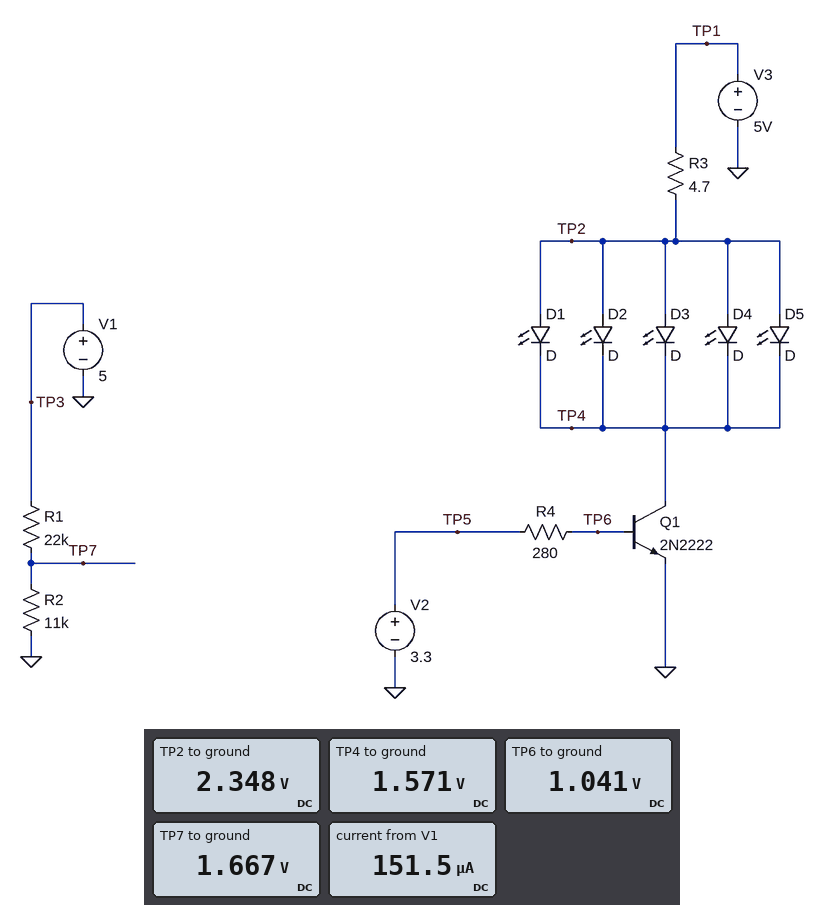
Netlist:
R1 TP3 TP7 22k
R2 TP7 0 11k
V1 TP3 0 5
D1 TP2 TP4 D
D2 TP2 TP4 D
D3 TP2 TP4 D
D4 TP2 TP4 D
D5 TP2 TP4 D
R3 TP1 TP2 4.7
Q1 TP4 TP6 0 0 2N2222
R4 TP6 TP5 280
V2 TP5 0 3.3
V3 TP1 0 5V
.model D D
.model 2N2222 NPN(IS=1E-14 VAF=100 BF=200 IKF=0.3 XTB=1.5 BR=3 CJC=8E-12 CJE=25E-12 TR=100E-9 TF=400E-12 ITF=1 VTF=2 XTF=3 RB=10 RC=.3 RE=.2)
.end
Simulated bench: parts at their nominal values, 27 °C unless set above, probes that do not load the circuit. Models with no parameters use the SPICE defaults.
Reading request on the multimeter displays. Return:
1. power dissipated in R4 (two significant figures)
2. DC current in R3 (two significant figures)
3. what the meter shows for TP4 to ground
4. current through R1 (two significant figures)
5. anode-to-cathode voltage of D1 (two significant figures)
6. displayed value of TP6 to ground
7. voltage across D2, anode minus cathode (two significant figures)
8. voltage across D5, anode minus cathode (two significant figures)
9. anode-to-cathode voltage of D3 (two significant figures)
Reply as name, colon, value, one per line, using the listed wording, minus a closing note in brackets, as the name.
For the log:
power dissipated in R4: 18 mW
DC current in R3: 560 mA
what the meter shows for TP4 to ground: 1.571 V
current through R1: 150 µA
anode-to-cathode voltage of D1: 780 mV
displayed value of TP6 to ground: 1.041 V
voltage across D2, anode minus cathode: 780 mV
voltage across D5, anode minus cathode: 780 mV
anode-to-cathode voltage of D3: 780 mV
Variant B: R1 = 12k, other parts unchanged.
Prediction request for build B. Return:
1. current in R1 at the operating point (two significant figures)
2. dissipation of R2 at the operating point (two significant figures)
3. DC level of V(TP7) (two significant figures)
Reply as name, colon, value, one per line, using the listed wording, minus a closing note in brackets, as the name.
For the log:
current in R1 at the operating point: 220 µA
dissipation of R2 at the operating point: 520 µW
DC level of V(TP7): 2.4 V
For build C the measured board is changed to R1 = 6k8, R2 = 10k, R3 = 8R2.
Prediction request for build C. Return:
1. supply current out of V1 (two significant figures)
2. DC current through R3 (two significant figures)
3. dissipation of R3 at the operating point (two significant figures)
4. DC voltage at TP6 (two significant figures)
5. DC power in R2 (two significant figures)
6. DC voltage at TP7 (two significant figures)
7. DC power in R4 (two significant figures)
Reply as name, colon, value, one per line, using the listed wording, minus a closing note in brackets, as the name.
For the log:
supply current out of V1: 300 µA
DC current through R3: 470 mA
dissipation of R3 at the operating point: 1.8 W
DC voltage at TP6: 1.0 V
DC power in R2: 890 µW
DC voltage at TP7: 3.0 V
DC power in R4: 19 mW
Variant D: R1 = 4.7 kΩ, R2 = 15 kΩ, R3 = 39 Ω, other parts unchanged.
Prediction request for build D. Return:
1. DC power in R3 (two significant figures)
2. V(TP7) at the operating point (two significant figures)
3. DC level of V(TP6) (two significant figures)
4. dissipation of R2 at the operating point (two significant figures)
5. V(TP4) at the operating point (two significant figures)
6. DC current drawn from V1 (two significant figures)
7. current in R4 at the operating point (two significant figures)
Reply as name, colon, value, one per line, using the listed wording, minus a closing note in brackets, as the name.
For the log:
DC power in R3: 440 mW
V(TP7) at the operating point: 3.8 V
DC level of V(TP6): 900 mV
dissipation of R2 at the operating point: 970 µW
V(TP4) at the operating point: 110 mV
DC current drawn from V1: 250 µA
current in R4 at the operating point: 8.6 mA
